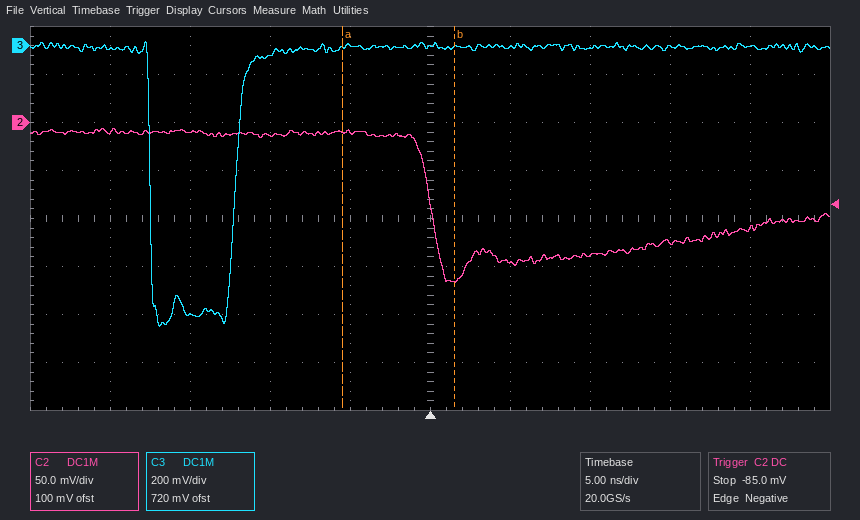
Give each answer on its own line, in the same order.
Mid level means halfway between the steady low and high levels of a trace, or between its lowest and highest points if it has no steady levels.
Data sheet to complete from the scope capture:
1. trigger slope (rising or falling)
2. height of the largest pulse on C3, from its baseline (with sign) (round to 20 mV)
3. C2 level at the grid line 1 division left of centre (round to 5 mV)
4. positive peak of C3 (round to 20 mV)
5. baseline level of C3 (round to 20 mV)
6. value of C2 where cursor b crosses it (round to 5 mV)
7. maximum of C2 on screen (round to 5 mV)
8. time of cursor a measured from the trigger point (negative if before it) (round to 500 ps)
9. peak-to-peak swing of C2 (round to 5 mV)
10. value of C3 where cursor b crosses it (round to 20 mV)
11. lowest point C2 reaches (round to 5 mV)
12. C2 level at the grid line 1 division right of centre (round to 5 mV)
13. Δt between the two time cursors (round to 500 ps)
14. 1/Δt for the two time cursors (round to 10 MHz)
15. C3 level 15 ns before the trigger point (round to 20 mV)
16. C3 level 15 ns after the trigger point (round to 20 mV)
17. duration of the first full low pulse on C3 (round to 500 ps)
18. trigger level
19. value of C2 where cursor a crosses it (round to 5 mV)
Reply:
falling
-1.16 V
-10 mV
20 mV
0 mV
-165 mV
-5 mV
-5.5 ns
160 mV
0 mV
-165 mV
-145 mV
7.0 ns
140 MHz
-1.12 V
0 mV
5.5 ns
-85.0 mV
-10 mV
